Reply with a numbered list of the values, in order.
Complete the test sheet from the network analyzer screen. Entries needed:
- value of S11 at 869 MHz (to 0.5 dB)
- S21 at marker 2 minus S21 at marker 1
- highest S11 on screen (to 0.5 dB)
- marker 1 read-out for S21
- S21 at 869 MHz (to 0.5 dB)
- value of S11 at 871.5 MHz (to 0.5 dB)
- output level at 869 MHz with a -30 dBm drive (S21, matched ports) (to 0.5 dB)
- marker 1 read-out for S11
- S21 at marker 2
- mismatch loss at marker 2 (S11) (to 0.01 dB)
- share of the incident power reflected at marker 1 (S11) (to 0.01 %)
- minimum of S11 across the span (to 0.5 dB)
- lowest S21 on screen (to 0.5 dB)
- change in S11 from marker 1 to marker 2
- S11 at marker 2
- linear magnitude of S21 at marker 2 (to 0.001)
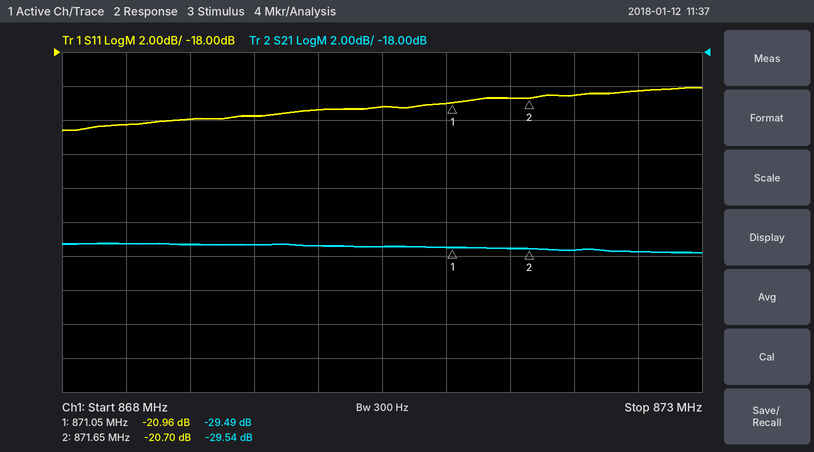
1. -22.0 dB
2. -0.05 dB
3. -20.0 dB
4. -29.49 dB
5. -29.5 dB
6. -20.5 dB
7. -59.5 dBm
8. -20.96 dB
9. -29.54 dB
10. 0.04 dB
11. 0.80 %
12. -22.5 dB
13. -30.0 dB
14. 0.26 dB
15. -20.70 dB
16. 0.033
